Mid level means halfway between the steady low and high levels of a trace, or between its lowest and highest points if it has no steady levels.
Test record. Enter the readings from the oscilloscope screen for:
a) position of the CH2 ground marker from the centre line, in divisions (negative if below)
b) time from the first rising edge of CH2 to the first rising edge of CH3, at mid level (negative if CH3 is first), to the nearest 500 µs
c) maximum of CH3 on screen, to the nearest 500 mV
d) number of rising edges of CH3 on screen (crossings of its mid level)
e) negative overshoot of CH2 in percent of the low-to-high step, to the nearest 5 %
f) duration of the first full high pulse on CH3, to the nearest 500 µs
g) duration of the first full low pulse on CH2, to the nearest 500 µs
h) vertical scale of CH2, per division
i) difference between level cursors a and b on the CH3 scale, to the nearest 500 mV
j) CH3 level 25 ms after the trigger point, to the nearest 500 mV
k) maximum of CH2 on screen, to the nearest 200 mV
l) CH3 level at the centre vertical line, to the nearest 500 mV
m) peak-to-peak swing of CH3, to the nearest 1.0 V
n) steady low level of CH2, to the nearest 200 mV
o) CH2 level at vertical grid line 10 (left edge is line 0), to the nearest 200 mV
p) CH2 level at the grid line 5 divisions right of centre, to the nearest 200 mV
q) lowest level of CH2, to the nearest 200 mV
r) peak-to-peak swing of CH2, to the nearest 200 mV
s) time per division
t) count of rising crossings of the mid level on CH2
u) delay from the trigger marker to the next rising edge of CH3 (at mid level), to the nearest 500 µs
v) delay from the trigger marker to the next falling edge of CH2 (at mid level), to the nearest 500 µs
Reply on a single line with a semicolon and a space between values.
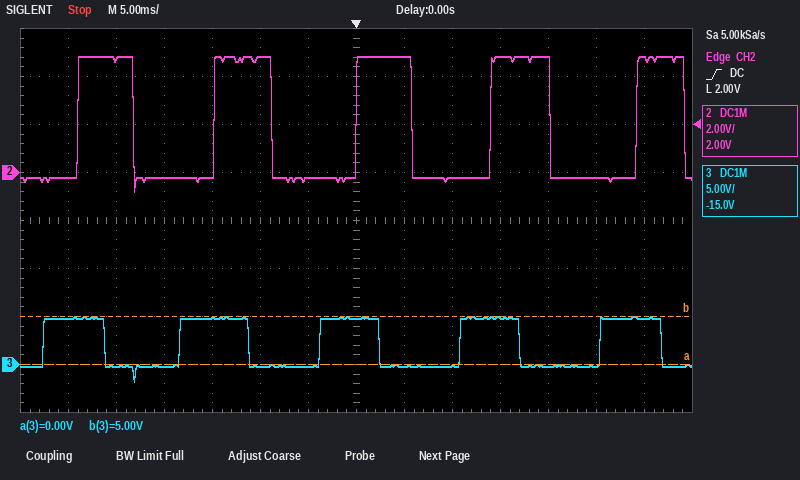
+1.0 div; -3.5 ms; 5.0 V; 5; 10 %; 6.5 ms; 8.5 ms; 2 V; 5.0 V; 0.0 V; 4.8 V; 5.0 V; 7.0 V; -200 mV; 4.8 V; -200 mV; -800 mV; 5.6 V; 5 ms; 5; 11.0 ms; 6.0 ms
